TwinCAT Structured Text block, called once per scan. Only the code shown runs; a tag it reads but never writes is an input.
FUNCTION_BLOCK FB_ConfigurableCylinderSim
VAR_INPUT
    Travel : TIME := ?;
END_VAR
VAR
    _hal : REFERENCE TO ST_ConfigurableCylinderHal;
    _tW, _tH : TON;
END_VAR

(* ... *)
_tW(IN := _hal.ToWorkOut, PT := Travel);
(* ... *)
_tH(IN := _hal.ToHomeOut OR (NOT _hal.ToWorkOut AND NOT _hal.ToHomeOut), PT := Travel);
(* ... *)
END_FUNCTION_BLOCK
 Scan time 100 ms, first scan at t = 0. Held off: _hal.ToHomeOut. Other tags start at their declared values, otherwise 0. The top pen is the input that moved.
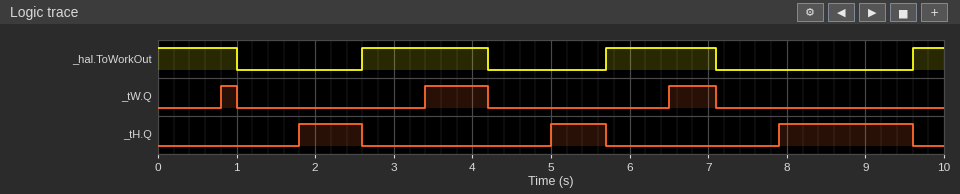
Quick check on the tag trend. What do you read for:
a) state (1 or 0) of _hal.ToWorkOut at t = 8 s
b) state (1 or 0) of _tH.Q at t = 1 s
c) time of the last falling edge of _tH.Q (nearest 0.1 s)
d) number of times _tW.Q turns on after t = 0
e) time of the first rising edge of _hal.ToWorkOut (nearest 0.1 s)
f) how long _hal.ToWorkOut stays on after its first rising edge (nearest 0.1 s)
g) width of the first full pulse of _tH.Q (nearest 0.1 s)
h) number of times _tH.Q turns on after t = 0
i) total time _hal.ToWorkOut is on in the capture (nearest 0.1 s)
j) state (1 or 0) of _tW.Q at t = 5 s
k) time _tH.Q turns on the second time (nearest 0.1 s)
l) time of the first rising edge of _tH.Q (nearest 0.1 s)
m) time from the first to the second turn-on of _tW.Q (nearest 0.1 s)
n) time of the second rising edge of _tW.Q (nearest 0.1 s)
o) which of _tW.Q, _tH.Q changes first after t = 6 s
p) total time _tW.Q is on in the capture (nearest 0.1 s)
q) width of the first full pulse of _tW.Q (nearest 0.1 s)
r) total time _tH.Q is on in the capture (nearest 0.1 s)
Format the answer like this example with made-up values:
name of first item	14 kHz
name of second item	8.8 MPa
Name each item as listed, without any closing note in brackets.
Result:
state (1 or 0) of _hal.ToWorkOut at t = 8 s	0
state (1 or 0) of _tH.Q at t = 1 s	0
time of the last falling edge of _tH.Q	9.6 s
number of times _tW.Q turns on after t = 0	3
time of the first rising edge of _hal.ToWorkOut	2.6 s
how long _hal.ToWorkOut stays on after its first rising edge	1.6 s
width of the first full pulse of _tH.Q	0.8 s
number of times _tH.Q turns on after t = 0	3
total time _hal.ToWorkOut is on in the capture	4.4 s
state (1 or 0) of _tW.Q at t = 5 s	0
time _tH.Q turns on the second time	5.0 s
time of the first rising edge of _tH.Q	1.8 s
time from the first to the second turn-on of _tW.Q	2.6 s
time of the second rising edge of _tW.Q	3.4 s
which of _tW.Q, _tH.Q changes first after t = 6 s	_tW.Q
total time _tW.Q is on in the capture	1.6 s
width of the first full pulse of _tW.Q	0.2 s
total time _tH.Q is on in the capture	3.2 s
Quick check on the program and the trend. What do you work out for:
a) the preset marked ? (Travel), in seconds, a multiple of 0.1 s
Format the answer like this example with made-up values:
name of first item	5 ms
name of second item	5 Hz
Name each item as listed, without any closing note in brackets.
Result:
the preset marked ? (Travel), in seconds, a multiple of 0.1 s	0.8 s
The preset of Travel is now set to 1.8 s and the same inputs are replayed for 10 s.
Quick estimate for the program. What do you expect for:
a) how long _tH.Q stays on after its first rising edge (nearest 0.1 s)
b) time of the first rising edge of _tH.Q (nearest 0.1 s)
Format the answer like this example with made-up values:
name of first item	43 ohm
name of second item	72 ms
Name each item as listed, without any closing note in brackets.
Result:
how long _tH.Q stays on after its first rising edge	0.7 s
time of the first rising edge of _tH.Q	8.9 s
